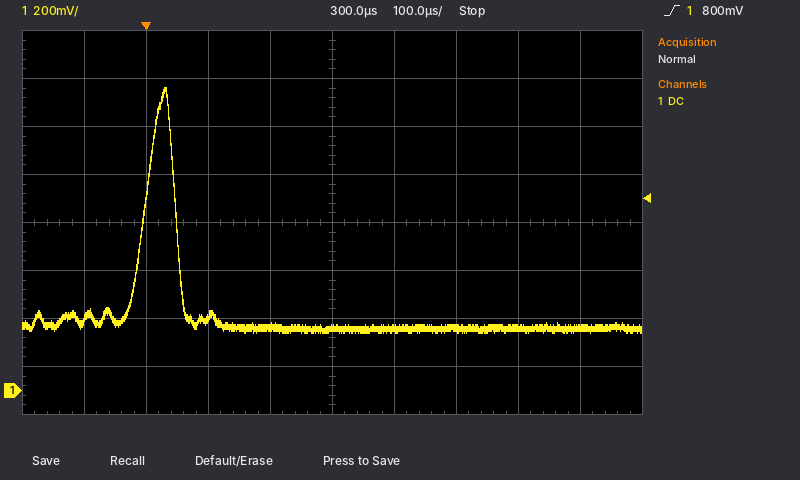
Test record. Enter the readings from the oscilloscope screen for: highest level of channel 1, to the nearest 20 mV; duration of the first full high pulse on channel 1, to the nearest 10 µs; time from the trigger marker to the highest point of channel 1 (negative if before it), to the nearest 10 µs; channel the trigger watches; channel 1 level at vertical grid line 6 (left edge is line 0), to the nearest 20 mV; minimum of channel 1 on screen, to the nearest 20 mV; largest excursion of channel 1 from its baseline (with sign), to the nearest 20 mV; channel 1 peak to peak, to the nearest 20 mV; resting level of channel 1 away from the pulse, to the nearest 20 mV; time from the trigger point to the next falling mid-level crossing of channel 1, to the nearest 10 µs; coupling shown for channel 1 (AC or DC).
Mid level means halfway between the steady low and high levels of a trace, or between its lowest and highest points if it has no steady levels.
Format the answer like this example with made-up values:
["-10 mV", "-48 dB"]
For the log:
["1.26 V", "50 µs", "+30 µs", "channel 1", "260 mV", "240 mV", "+1.00 V", "1.02 V", "260 mV", "50 µs", "DC"]
